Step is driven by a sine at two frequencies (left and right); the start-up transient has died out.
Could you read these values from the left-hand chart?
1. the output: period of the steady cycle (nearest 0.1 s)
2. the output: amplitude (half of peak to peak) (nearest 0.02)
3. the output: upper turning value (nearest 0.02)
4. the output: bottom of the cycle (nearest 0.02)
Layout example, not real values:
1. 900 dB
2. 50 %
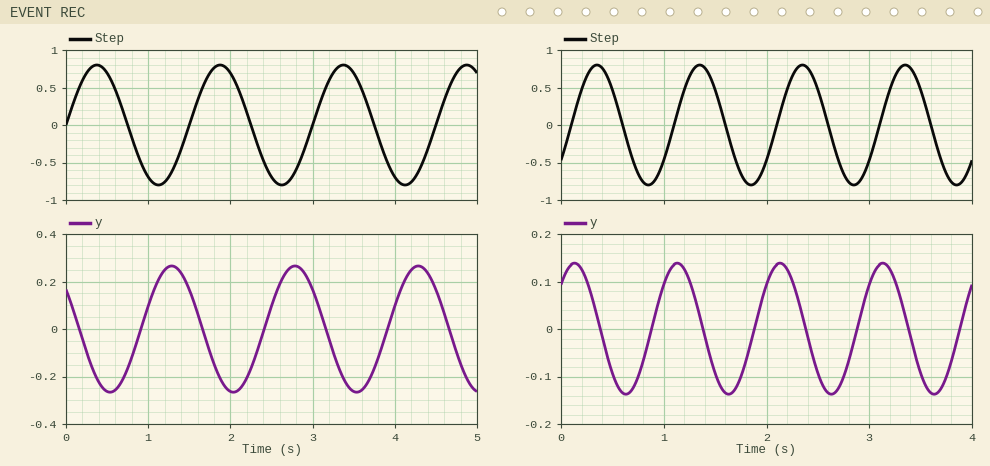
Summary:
1. 1.5 s
2. 0.26
3. 0.26
4. -0.26
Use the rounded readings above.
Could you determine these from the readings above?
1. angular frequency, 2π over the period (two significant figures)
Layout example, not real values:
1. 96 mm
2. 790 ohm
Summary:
1. 4.2 rad/s
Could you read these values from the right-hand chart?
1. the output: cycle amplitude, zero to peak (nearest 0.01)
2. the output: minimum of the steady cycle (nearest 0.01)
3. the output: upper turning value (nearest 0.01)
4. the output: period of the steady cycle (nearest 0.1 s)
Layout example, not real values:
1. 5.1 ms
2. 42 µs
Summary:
1. 0.14
2. -0.14
3. 0.14
4. 1.0 s
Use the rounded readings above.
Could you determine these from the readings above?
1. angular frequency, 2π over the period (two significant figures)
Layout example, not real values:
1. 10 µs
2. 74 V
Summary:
1. 6.3 rad/s
